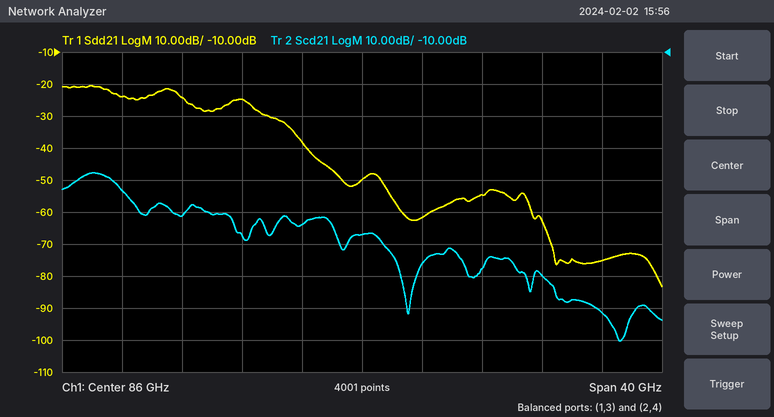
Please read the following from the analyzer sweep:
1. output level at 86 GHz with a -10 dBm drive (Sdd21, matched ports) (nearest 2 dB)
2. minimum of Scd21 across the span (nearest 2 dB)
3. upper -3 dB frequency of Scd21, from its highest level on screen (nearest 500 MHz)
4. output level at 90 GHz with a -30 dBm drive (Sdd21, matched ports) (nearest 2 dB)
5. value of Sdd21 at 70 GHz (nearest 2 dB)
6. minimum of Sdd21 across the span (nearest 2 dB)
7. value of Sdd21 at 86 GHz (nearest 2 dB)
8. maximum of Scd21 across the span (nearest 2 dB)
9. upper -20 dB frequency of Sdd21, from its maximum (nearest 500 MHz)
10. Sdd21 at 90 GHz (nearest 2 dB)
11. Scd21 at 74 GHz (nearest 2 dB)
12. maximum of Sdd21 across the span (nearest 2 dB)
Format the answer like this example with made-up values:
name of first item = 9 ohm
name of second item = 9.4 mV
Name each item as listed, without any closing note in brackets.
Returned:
output level at 86 GHz with a -10 dBm drive (Sdd21, matched ports) = -60 dBm
minimum of Scd21 across the span = -100 dB
upper -3 dB frequency of Scd21, from its highest level on screen = 69.5 GHz
output level at 90 GHz with a -30 dBm drive (Sdd21, matched ports) = -92 dBm
value of Sdd21 at 70 GHz = -24 dB
minimum of Sdd21 across the span = -84 dB
value of Sdd21 at 86 GHz = -50 dB
maximum of Scd21 across the span = -48 dB
upper -20 dB frequency of Sdd21, from its maximum = 82.5 GHz
Sdd21 at 90 GHz = -62 dB
Scd21 at 74 GHz = -62 dB
maximum of Sdd21 across the span = -20 dB
